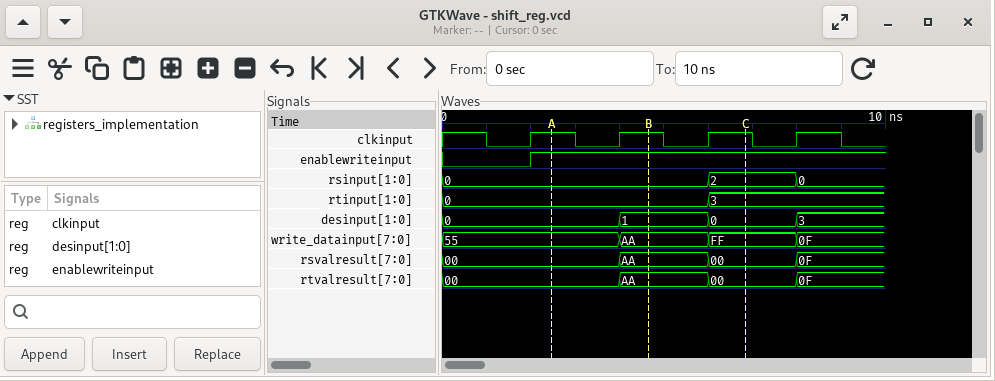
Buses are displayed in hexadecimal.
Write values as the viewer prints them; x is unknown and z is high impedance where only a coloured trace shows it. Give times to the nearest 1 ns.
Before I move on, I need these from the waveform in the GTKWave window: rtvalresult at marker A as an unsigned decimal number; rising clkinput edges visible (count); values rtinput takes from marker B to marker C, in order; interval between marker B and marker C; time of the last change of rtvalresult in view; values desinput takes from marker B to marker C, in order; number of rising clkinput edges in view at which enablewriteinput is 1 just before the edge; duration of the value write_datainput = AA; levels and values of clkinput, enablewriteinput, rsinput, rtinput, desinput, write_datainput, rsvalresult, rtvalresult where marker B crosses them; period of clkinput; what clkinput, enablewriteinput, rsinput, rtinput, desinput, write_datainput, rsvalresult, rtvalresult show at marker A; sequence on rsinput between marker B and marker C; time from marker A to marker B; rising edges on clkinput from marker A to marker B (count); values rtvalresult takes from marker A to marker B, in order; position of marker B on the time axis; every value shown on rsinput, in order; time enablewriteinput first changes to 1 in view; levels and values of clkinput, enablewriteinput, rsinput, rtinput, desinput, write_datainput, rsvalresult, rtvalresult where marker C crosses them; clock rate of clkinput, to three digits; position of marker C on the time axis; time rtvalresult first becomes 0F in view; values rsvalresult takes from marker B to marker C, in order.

0
4
0, 3
2 ns
8 ns
1, 0
3
2 ns
clkinput=1, enablewriteinput=1, rsinput=0, rtinput=0, desinput=1, write_datainput=AA, rsvalresult=AA, rtvalresult=AA
2 ns
clkinput=1, enablewriteinput=1, rsinput=0, rtinput=0, desinput=0, write_datainput=55, rsvalresult=00, rtvalresult=00
0, 2
2 ns
1
00, AA
5 ns
0, 2, 0
2 ns
clkinput=1, enablewriteinput=1, rsinput=2, rtinput=3, desinput=0, write_datainput=FF, rsvalresult=00, rtvalresult=00
500 MHz
7 ns
8 ns
AA, 00
